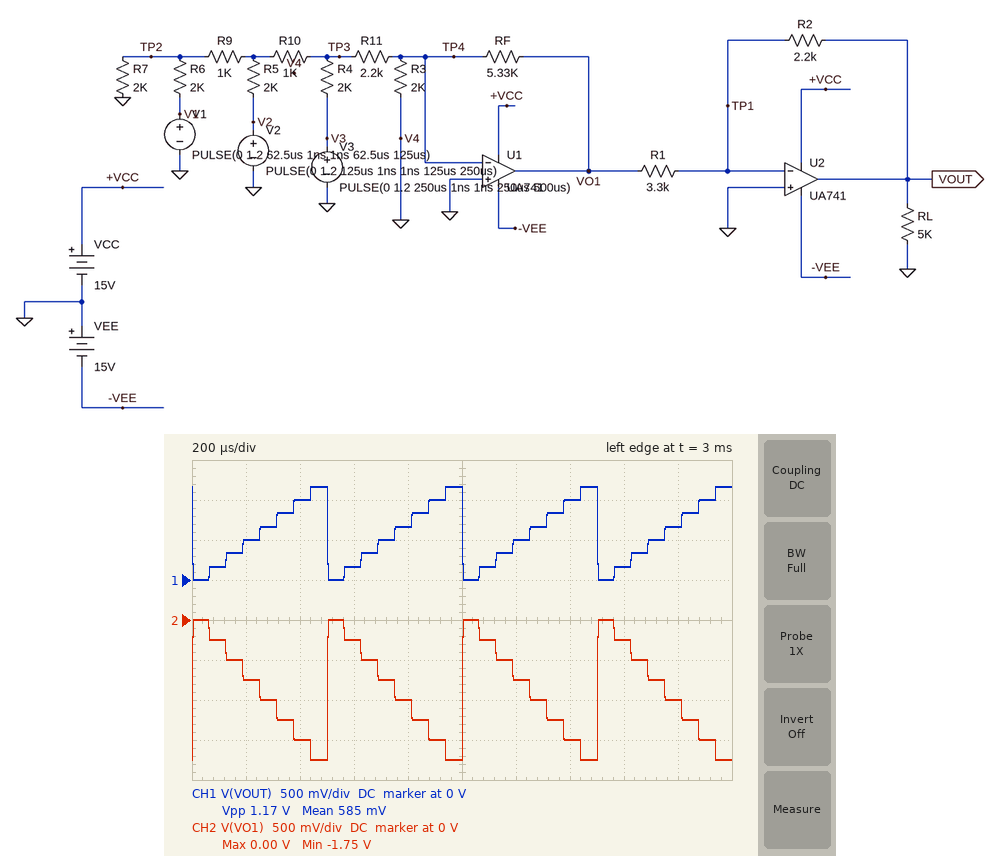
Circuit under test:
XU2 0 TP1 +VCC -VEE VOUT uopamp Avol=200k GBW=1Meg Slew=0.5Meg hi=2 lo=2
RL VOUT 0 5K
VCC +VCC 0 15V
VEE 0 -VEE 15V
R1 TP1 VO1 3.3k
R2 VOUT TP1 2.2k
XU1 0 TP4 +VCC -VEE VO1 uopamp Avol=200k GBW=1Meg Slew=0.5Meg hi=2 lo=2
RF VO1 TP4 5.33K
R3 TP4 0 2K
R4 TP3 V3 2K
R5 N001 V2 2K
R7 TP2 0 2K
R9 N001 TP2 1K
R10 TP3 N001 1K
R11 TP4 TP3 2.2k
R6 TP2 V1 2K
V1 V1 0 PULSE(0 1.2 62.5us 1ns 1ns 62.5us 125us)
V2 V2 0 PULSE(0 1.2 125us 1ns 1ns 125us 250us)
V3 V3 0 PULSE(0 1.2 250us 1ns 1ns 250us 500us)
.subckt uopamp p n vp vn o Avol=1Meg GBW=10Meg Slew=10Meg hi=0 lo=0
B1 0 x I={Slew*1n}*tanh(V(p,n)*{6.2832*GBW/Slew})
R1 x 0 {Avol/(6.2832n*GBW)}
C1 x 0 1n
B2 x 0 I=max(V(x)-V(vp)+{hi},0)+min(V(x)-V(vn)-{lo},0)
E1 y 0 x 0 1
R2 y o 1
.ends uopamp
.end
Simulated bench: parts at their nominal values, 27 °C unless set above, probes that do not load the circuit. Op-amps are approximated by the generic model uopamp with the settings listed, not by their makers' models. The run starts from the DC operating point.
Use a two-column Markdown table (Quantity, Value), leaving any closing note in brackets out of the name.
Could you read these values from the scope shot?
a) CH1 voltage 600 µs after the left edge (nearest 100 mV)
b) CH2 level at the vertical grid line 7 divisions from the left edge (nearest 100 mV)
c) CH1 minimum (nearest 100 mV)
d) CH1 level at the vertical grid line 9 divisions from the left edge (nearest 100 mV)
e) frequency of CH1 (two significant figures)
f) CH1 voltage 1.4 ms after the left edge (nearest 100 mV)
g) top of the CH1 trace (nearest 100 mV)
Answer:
| Quantity | Value |
|---|---|
| CH1 voltage 600 µs after the left edge | 200 mV |
| CH2 level at the vertical grid line 7 divisions from the left edge | -1.5 V |
| CH1 minimum | 0 V |
| CH1 level at the vertical grid line 9 divisions from the left edge | 700 mV |
| frequency of CH1 | 2.0 kHz |
| CH1 voltage 1.4 ms after the left edge | 1.0 V |
| top of the CH1 trace | 1.2 V |
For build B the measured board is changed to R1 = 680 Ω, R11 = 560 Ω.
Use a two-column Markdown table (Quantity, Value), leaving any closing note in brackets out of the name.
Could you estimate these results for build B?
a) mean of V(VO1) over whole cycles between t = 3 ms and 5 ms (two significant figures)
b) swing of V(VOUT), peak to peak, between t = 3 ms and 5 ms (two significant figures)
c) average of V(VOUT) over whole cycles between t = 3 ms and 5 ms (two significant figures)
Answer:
| Quantity | Value |
|---|---|
| mean of V(VO1) over whole cycles between t = 3 ms and 5 ms | -1.8 V |
| swing of V(VOUT), peak to peak, between t = 3 ms and 5 ms | 12 V |
| average of V(VOUT) over whole cycles between t = 3 ms and 5 ms | 6.0 V |
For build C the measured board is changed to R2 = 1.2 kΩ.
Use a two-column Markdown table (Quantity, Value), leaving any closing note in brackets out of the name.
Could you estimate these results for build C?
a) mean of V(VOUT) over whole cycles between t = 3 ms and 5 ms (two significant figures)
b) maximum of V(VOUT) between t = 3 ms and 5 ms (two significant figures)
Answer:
| Quantity | Value |
|---|---|
| mean of V(VOUT) over whole cycles between t = 3 ms and 5 ms | 320 mV |
| maximum of V(VOUT) between t = 3 ms and 5 ms | 640 mV |
